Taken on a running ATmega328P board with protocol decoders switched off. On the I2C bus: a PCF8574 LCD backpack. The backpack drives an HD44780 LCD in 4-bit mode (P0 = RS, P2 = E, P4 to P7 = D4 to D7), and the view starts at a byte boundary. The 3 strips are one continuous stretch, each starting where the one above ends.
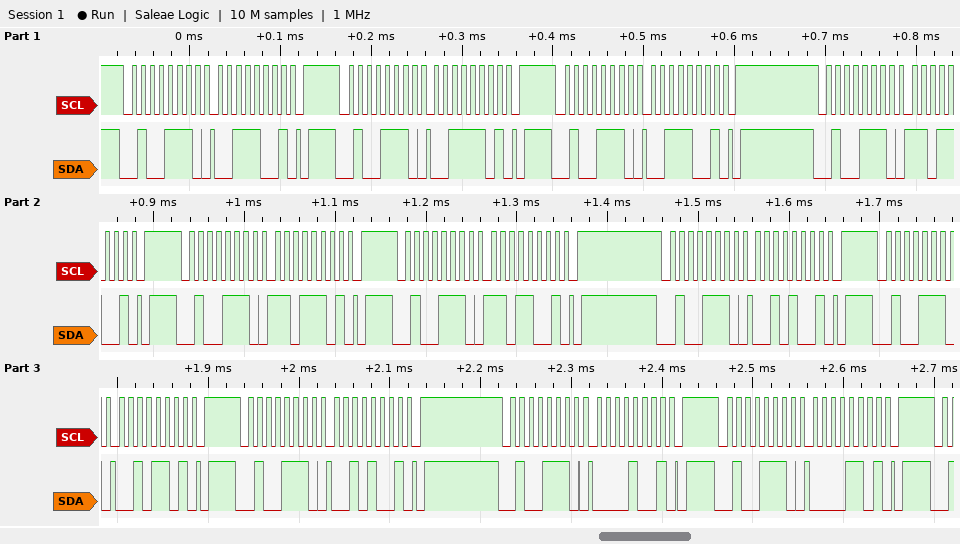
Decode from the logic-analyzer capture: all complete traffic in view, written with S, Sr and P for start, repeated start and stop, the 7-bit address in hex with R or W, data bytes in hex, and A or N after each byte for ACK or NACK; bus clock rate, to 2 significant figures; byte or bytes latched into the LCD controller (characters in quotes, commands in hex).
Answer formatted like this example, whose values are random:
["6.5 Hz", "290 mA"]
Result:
["S 27W A 39 A P S 27W A 3D A P S 27W A 39 A P S 27W A D9 A P S 27W A DD A P S 27W A D9 A P S 27W A 29 A P S 27W A 2D A P S 27W A 29 A P S 27W A 09 A P S 27W A 0D A P", "100 kHz", "'='"]
